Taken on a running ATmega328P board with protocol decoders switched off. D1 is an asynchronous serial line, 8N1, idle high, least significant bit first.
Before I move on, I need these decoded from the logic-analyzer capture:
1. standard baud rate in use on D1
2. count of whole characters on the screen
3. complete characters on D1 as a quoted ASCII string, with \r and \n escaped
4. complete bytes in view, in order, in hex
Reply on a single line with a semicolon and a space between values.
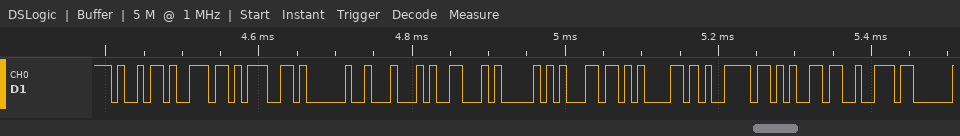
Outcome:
115200 baud; 12; "ing DFPlayer"; 0x69 0x6E 0x67 0x20 0x44 0x46 0x50 0x6C 0x61 0x79 0x65 0x72
